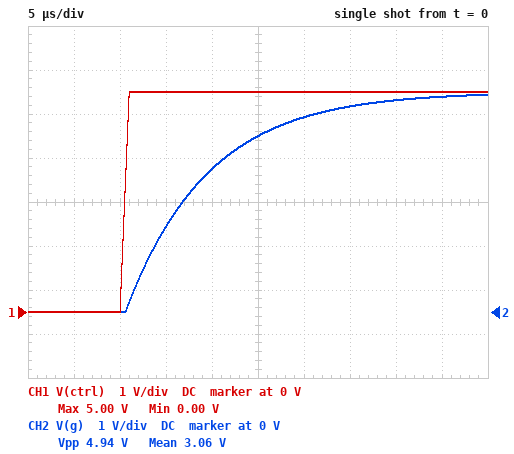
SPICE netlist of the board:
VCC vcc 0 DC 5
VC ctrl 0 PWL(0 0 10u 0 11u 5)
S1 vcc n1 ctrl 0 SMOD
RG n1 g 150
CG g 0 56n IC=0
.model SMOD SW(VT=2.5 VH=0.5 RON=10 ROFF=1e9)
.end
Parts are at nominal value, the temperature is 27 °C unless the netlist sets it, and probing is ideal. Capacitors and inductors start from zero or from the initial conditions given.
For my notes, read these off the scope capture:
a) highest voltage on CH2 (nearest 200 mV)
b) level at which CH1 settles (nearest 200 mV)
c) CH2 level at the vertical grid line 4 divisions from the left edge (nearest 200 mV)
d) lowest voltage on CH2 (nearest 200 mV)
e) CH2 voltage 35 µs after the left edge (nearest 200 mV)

5.0 V
5.0 V
3.2 V
0 V
4.6 V
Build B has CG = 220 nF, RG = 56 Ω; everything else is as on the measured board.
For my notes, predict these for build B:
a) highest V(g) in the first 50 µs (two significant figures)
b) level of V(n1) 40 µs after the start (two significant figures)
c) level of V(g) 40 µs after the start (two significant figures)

4.7 V
4.9 V
4.3 V
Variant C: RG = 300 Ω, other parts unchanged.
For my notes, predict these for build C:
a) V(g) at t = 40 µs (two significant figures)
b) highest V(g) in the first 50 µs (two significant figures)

4.1 V
4.5 V
